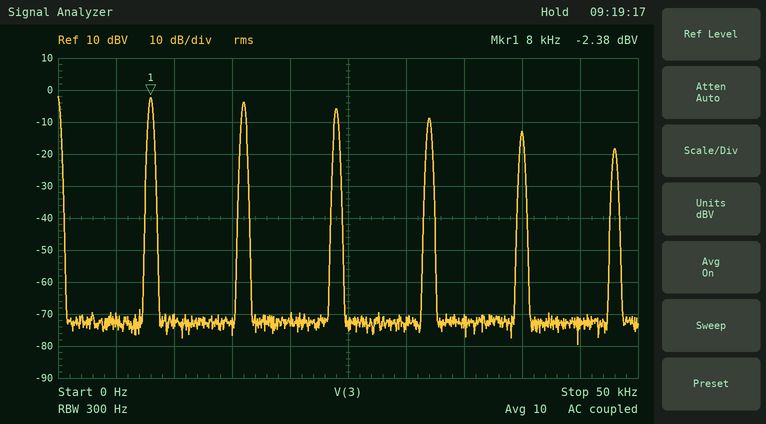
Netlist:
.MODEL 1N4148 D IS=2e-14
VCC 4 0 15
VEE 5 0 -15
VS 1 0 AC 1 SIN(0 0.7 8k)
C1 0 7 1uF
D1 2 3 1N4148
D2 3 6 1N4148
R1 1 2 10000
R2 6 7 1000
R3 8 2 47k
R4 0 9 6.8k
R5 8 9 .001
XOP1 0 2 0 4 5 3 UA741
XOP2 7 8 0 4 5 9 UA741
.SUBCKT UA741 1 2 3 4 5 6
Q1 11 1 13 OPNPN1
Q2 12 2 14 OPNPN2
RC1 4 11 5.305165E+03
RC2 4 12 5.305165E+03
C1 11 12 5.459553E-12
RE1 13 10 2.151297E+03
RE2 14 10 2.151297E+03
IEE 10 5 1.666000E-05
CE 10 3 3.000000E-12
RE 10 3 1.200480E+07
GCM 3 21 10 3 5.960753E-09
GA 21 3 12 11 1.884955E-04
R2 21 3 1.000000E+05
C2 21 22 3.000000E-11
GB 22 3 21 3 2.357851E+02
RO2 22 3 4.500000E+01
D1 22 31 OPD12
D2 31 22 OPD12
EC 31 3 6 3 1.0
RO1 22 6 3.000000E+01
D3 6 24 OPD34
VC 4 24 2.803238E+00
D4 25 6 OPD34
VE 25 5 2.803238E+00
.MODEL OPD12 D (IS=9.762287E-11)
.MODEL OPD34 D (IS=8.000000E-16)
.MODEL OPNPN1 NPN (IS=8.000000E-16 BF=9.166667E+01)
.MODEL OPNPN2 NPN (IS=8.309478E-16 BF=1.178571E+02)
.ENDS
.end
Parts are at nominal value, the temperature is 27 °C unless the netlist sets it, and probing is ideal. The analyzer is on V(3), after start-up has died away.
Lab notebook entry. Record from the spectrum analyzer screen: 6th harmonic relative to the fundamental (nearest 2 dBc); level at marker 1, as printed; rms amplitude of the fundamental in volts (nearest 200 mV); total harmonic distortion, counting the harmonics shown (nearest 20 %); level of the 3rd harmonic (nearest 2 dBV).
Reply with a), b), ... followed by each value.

a) -16 dBc
b) -2.38 dBV
c) 800 mV
d) 120 %
e) -6 dBV
